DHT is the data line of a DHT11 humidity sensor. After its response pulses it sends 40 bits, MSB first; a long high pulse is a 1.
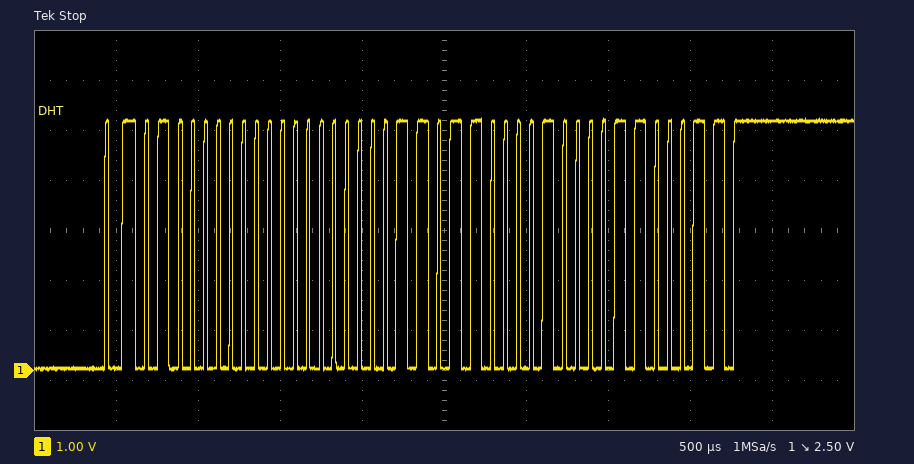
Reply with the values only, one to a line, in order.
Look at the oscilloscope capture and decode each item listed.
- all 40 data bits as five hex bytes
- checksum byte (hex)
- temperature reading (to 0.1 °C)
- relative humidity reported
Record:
40 00 1B 08 63
0x63
27.8 °C
64 %
